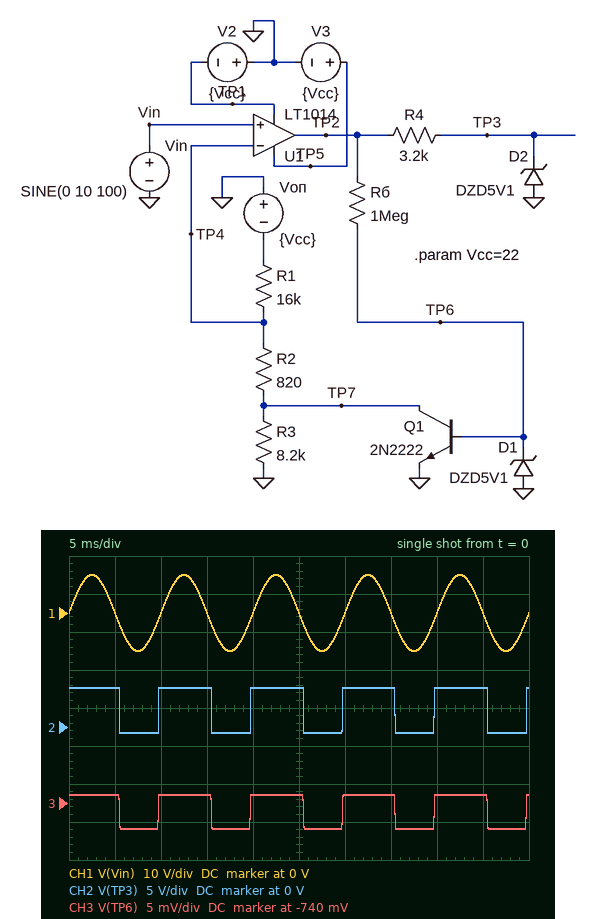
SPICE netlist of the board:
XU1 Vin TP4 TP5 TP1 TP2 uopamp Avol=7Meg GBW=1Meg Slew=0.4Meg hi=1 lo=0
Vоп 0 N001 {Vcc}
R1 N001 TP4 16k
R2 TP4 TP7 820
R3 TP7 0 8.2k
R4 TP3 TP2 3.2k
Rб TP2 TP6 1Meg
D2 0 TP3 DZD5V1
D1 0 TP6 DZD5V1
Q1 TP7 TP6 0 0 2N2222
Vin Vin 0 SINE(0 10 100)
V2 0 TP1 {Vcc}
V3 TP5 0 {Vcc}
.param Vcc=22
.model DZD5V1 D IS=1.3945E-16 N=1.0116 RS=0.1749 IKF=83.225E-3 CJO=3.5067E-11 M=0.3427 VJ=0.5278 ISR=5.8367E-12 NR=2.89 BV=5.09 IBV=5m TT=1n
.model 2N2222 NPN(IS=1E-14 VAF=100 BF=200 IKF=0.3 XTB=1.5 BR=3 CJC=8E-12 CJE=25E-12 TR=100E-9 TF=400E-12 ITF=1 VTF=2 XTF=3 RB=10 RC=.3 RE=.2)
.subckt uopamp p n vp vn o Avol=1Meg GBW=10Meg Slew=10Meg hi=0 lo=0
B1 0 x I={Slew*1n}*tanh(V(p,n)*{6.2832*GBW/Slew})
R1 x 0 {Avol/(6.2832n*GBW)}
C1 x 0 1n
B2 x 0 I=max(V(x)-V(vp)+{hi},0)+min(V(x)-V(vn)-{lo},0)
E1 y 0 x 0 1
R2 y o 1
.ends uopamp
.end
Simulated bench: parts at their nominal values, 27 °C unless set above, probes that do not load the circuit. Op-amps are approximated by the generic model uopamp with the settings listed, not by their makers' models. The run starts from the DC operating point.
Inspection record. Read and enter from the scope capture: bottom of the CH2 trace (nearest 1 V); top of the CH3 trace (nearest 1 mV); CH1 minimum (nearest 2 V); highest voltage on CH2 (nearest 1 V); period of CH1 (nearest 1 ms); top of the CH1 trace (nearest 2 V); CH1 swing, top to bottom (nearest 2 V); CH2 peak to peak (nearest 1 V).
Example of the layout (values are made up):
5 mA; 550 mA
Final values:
-1 V; -739 mV; -10 V; 5 V; 10 ms; 10 V; 20 V; 6 V
